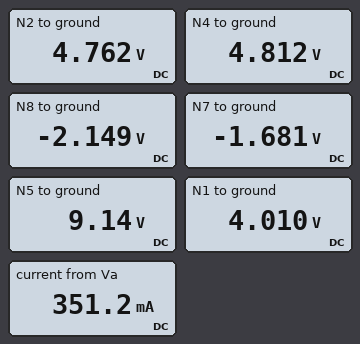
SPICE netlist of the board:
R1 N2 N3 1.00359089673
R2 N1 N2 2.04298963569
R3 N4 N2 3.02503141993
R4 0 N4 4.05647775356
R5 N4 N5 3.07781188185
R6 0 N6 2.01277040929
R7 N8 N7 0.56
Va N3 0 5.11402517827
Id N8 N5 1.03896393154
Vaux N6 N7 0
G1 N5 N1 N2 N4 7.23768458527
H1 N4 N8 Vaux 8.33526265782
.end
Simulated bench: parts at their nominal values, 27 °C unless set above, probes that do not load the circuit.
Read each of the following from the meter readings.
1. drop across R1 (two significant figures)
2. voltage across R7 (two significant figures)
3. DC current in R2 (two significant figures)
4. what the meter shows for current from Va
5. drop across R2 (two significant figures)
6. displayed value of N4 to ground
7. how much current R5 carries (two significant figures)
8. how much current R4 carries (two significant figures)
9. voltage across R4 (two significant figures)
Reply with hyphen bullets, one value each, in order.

- 350 mV
- 470 mV
- 370 mA
- 351.2 mA
- 750 mV
- 4.812 V
- 1.4 A
- 1.2 A
- 4.8 V
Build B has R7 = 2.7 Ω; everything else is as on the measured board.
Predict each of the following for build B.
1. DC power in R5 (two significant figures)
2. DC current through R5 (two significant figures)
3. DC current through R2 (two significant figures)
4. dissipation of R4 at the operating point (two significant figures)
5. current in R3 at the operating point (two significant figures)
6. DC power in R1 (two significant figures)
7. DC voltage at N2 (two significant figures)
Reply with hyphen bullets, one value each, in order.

- 2.4 W
- 880 mA
- 160 mA
- 6.8 W
- 7.4 mA
- 24 mW
- 5.3 V
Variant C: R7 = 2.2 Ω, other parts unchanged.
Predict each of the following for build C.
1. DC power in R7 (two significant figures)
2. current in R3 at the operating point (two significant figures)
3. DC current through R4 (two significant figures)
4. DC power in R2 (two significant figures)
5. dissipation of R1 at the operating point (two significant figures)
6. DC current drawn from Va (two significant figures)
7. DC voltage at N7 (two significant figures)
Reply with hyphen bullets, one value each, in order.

- 3.4 W
- 960 µA
- 1.3 A
- 910 µW
- 410 µW
- 20 mA
- -2.5 V
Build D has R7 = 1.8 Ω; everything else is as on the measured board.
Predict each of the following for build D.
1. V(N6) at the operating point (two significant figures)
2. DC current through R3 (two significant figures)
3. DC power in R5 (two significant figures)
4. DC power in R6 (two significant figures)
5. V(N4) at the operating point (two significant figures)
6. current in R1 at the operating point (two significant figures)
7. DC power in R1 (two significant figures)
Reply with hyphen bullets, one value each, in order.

- -2.2 V
- 6.1 mA
- 4.2 W
- 2.5 W
- 5.0 V
- 130 mA
- 16 mW
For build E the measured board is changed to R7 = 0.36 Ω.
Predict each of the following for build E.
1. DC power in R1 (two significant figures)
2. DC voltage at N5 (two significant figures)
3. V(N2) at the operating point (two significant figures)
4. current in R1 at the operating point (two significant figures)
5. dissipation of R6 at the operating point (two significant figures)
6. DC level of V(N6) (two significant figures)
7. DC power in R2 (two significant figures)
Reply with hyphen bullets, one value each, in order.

- 140 mW
- 9.2 V
- 4.7 V
- 380 mA
- 1.3 W
- -1.6 V
- 320 mW
